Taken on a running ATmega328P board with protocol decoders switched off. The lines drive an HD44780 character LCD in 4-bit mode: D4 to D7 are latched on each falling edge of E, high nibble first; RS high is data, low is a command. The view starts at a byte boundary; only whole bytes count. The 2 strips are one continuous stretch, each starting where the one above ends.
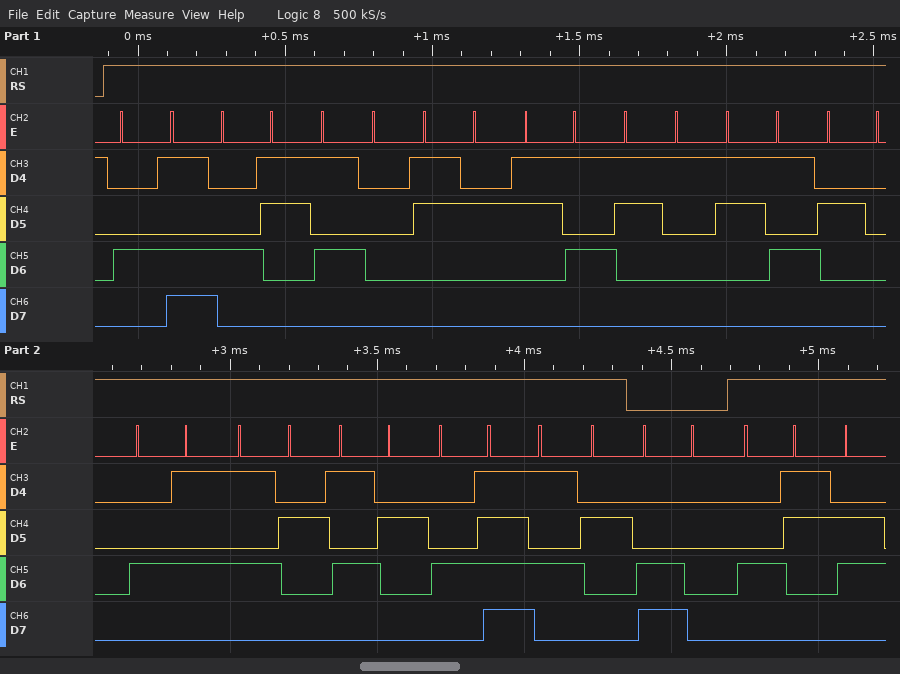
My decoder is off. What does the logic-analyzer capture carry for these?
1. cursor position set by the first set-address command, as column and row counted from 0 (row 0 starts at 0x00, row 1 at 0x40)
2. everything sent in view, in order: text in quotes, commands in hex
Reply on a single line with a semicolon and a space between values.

column 0, row 1; "MCP2515 ERROR" 0xC0 "C"
